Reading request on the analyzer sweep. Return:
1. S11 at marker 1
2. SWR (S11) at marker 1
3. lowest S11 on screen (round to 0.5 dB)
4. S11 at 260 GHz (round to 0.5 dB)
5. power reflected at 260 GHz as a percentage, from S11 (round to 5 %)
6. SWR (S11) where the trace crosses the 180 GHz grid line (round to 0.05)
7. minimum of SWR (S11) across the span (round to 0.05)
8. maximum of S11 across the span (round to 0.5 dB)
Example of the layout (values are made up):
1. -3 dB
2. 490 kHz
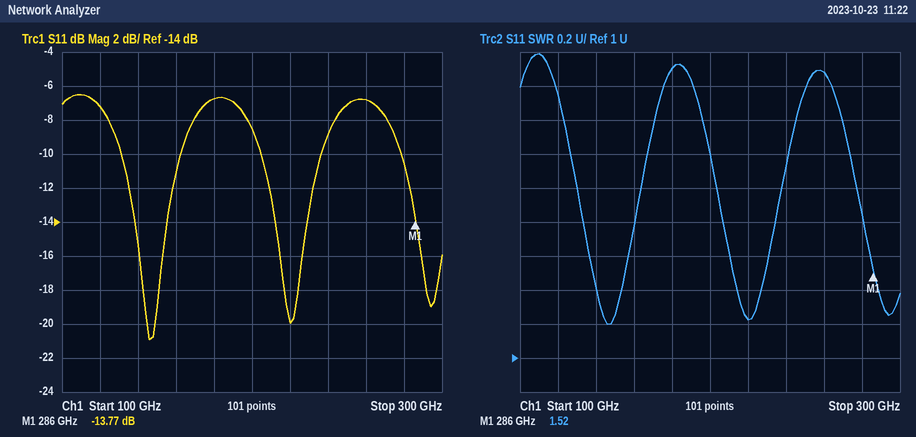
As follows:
1. -13.77 dB
2. 1.52
3. -21.0 dB
4. -7.0 dB
5. 20 %
6. 2.70
7. 1.20
8. -6.5 dB
